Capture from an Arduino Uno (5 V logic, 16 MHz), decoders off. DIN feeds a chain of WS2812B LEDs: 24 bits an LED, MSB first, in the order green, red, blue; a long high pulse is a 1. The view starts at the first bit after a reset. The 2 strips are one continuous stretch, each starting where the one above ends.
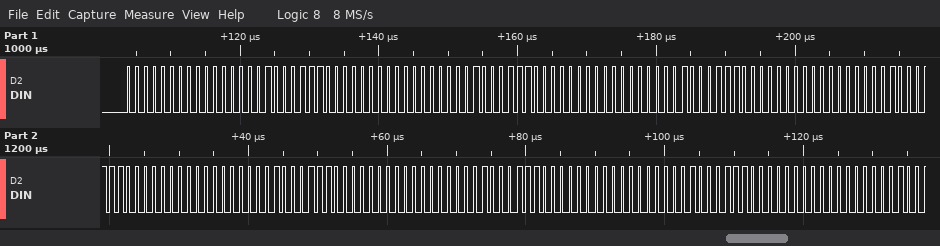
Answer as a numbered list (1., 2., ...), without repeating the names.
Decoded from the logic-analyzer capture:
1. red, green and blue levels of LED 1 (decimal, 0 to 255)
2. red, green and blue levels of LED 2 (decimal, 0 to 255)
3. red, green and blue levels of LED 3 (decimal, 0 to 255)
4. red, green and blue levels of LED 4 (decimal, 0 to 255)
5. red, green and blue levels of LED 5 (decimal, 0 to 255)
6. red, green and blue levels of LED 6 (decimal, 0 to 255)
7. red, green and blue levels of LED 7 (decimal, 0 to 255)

1. 0, 0, 142
2. 0, 0, 142
3. 0, 0, 142
4. 0, 0, 142
5. 0, 0, 142
6. 0, 0, 142
7. 0, 0, 142
